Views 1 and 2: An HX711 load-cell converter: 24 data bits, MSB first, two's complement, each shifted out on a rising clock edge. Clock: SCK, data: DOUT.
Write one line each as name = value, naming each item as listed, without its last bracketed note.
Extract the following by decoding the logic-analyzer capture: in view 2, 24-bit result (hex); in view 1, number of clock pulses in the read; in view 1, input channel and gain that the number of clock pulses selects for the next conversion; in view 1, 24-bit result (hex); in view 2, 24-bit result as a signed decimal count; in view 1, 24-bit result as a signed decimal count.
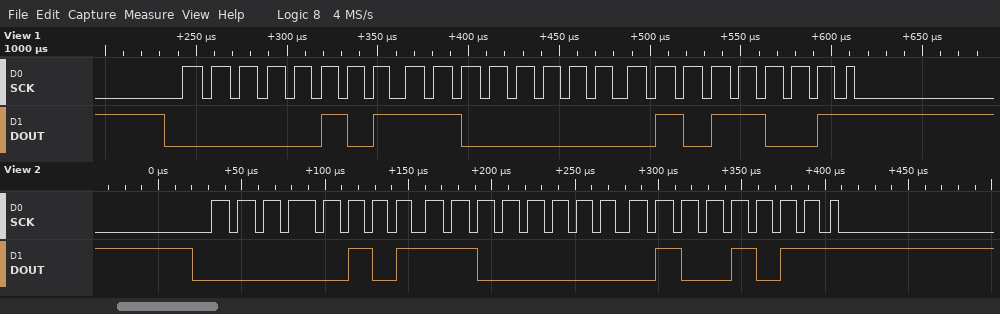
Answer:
in view 2, 24-bit result = 0x05C04B
in view 1, number of clock pulses in the read = 25
in view 1, input channel and gain that the number of clock pulses selects for the next conversion = channel A, gain 128
in view 1, 24-bit result = 0x05C059
in view 2, 24-bit result as a signed decimal count = 376907
in view 1, 24-bit result as a signed decimal count = 376921
